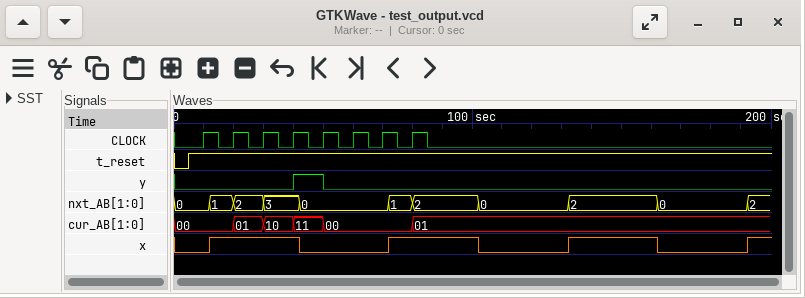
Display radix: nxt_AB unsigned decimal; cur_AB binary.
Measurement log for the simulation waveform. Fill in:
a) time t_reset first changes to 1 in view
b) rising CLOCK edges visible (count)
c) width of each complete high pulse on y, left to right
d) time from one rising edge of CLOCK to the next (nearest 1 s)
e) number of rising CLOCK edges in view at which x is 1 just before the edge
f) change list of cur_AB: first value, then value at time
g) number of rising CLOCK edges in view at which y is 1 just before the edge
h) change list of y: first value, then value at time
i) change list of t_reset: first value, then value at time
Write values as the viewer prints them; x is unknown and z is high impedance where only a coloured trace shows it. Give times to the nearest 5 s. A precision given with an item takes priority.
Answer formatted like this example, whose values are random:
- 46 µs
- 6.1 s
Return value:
- 5 s
- 8
- 10 s
- 10 s
- 4
- 00, 01 at 20 s, 10 at 30 s, 11 at 40 s, 00 at 50 s, 01 at 80 s
- 1
- 0, 1 at 40 s, 0 at 50 s
- 0, 1 at 5 s
